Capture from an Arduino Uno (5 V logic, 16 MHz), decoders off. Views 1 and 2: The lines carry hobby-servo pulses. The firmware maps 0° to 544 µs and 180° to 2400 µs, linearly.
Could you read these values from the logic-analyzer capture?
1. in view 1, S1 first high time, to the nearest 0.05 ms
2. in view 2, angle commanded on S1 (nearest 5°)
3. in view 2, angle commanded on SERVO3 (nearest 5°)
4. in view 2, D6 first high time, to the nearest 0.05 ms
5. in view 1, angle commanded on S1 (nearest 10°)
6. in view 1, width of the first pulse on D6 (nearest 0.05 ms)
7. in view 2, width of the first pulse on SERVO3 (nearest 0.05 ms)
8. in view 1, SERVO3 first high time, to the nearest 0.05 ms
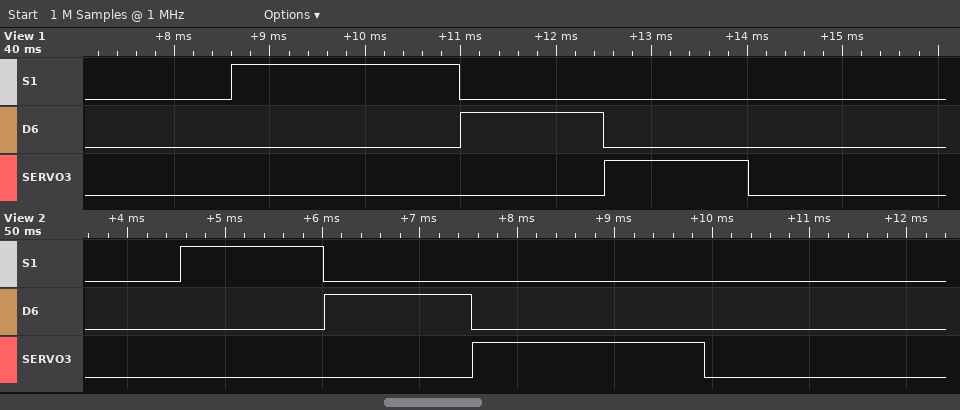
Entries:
2.40 ms
90°
180°
1.50 ms
180°
1.50 ms
2.40 ms
1.50 ms
